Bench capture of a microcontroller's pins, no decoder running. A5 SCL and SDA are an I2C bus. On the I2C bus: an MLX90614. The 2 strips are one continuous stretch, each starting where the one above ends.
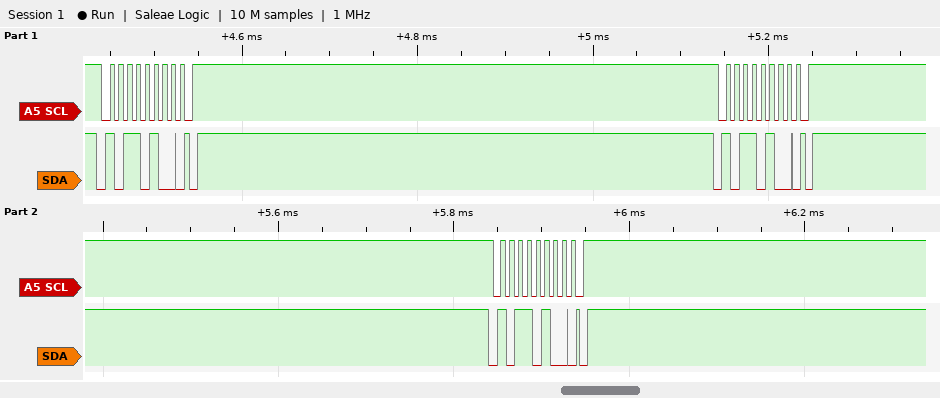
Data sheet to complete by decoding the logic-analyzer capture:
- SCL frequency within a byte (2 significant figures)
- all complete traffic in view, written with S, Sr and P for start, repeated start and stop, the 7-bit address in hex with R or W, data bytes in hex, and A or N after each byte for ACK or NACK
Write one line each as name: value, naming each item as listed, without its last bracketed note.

SCL frequency within a byte: 100 kHz
all complete traffic in view, written with S, Sr and P for start, repeated start and stop, the 7-bit address in hex with R or W, data bytes in hex, and A or N after each byte for ACK or NACK: S 5AW A P S 5AW A P S 5AW A P
